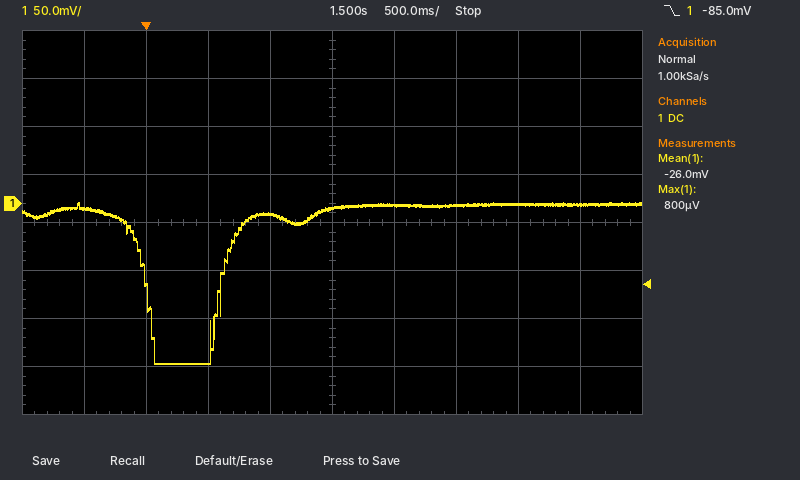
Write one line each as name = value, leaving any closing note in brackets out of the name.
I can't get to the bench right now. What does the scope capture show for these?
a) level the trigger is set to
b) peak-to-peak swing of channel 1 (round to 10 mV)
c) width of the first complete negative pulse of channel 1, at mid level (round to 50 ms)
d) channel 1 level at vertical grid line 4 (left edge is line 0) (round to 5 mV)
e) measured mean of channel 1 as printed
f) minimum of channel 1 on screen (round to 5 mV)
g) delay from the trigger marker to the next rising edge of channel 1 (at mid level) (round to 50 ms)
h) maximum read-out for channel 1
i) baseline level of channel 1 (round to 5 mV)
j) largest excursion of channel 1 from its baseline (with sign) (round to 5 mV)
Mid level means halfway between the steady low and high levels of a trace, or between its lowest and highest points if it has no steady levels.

level the trigger is set to = -85.0 mV
peak-to-peak swing of channel 1 = 170 mV
width of the first complete negative pulse of channel 1, at mid level = 600 ms
channel 1 level at vertical grid line 4 (left edge is line 0) = -10 mV
measured mean of channel 1 as printed = -26.0 mV
minimum of channel 1 on screen = -165 mV
delay from the trigger marker to the next rising edge of channel 1 (at mid level) = 600 ms
maximum read-out for channel 1 = 800 µV
baseline level of channel 1 = 0 mV
largest excursion of channel 1 from its baseline (with sign) = -165 mV
